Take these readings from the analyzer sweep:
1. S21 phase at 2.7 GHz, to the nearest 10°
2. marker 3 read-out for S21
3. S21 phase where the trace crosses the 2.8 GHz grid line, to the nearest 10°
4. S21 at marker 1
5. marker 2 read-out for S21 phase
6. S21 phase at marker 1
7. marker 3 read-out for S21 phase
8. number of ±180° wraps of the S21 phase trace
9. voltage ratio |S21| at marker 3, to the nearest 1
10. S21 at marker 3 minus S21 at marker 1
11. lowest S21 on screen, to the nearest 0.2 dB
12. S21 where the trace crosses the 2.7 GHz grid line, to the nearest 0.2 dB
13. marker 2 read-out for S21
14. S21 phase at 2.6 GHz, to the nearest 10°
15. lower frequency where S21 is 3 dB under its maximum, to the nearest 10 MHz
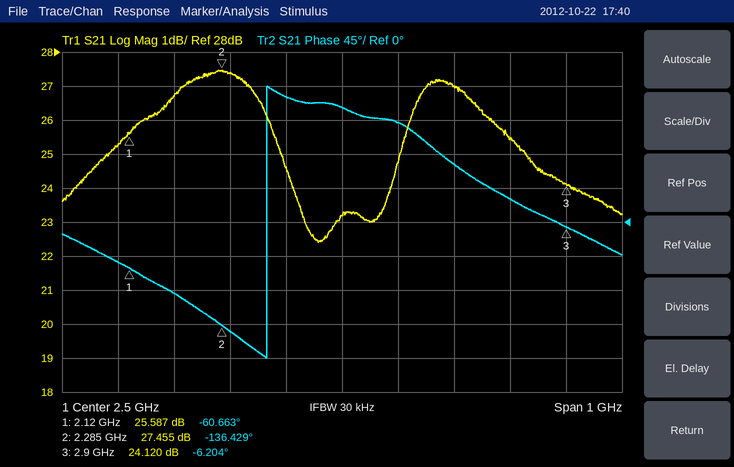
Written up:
80°
24.120 dB
30°
25.587 dB
-136.429°
-60.663°
-6.204°
1
16
-1.467 dB
22.4 dB
27.0 dB
27.455 dB
130°
2.05 GHz
